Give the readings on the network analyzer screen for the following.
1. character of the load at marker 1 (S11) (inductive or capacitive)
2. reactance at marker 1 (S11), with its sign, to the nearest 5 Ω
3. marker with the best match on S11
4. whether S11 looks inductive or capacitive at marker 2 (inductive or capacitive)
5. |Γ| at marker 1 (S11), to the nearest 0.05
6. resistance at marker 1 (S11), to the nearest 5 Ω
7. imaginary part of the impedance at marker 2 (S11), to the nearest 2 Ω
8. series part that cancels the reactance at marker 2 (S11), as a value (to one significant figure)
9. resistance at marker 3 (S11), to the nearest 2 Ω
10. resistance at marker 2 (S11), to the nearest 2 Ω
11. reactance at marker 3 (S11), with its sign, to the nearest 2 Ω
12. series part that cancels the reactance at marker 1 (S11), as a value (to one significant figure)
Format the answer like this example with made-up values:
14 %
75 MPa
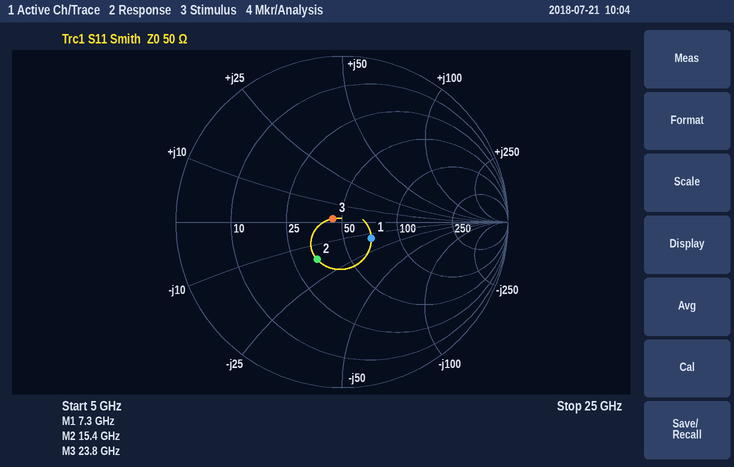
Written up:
capacitive
-15 Ω
marker 3
capacitive
0.20
70 Ω
-16 Ω
200 pH
44 Ω
34 Ω
+2 Ω
300 pH
